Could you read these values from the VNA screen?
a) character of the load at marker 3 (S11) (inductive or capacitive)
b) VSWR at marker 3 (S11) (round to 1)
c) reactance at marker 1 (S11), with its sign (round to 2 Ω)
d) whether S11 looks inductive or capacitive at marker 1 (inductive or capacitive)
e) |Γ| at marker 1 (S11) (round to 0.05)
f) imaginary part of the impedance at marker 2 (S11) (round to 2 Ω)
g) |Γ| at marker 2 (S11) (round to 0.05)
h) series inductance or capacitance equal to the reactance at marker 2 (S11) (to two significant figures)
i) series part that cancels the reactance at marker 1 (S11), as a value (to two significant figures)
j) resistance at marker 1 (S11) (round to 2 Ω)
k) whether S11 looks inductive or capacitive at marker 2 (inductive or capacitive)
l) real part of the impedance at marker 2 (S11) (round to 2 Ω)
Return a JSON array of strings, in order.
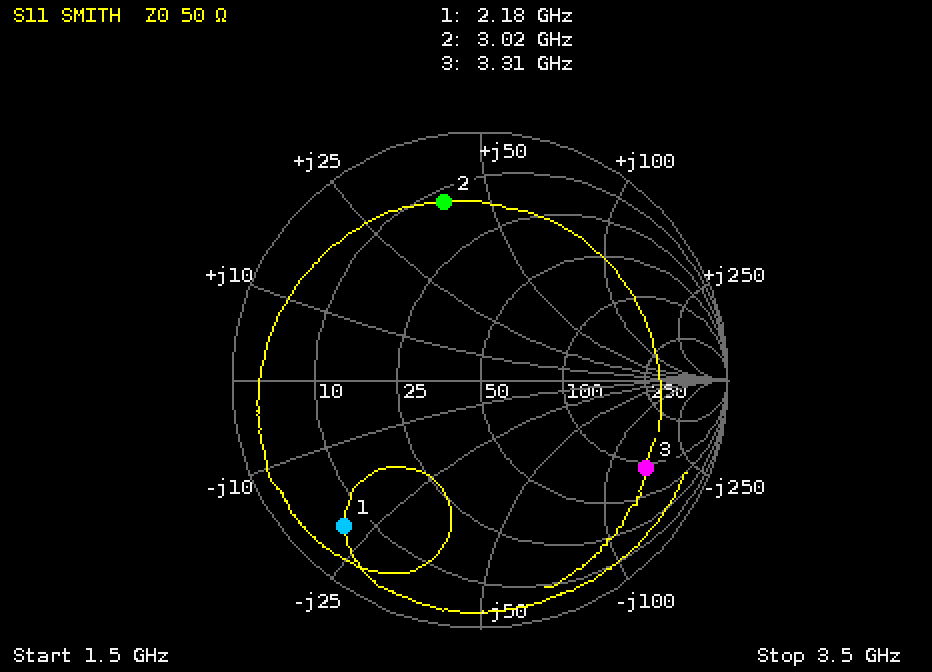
["capacitive", "7", "-22 Ω", "capacitive", "0.80", "+40 Ω", "0.75", "2.1 nH", "1.6 nH", "6 Ω", "inductive", "12 Ω"]
